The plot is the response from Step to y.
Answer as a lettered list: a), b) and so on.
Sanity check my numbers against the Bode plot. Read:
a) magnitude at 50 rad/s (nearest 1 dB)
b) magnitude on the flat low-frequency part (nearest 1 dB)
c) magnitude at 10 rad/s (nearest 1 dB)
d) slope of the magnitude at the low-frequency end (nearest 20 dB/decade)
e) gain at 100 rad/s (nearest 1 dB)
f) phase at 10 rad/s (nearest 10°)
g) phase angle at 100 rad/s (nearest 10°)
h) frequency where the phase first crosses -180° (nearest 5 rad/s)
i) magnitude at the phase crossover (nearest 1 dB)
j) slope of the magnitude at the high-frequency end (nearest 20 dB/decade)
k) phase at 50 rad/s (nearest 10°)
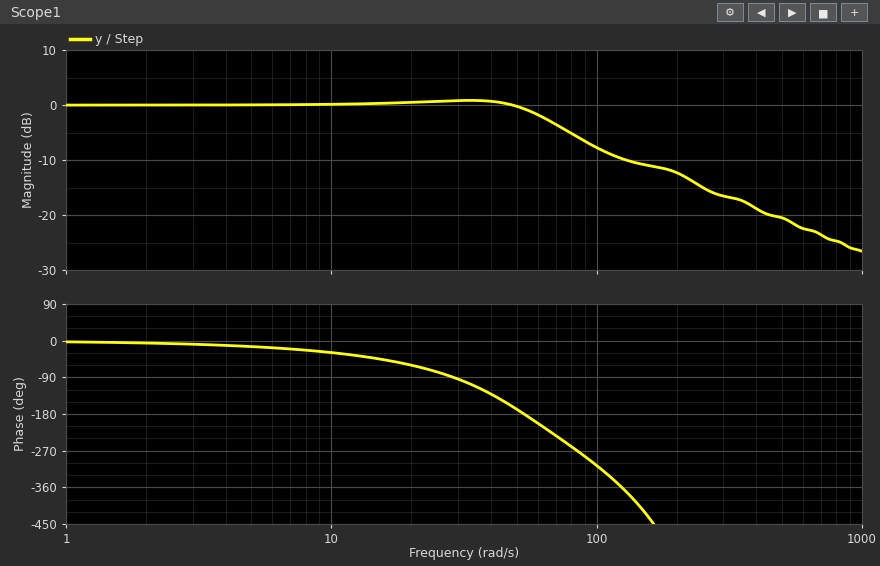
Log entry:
a) 0 dB
b) 0 dB
c) 0 dB
d) 0 dB/decade
e) -8 dB
f) -30°
g) -310°
h) 55 rad/s
i) -1 dB
j) -20 dB/decade
k) -170°
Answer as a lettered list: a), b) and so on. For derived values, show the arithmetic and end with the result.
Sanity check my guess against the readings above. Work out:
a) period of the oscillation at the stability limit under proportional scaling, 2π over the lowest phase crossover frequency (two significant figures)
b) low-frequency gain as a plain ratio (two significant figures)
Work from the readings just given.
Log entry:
a) 2π / 55 = 0.11 s
b) 10^(0 / 20) = 1.0
